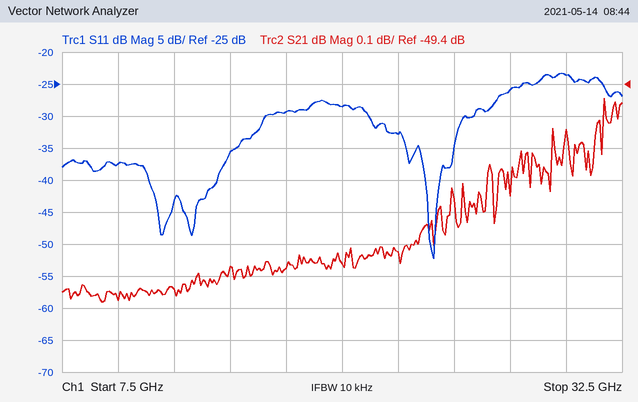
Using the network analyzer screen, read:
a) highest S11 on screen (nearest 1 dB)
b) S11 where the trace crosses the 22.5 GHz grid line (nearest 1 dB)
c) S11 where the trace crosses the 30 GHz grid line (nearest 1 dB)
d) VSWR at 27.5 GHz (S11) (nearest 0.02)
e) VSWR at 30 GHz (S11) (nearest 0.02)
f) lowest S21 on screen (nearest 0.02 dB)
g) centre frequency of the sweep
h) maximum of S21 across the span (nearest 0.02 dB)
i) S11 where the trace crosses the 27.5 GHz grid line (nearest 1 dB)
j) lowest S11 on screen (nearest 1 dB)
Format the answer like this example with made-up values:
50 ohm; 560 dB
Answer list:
-23 dB; -33 dB; -24 dB; 1.10; 1.14; -50.08 dB; 20 GHz; -49.44 dB; -26 dB; -52 dB
